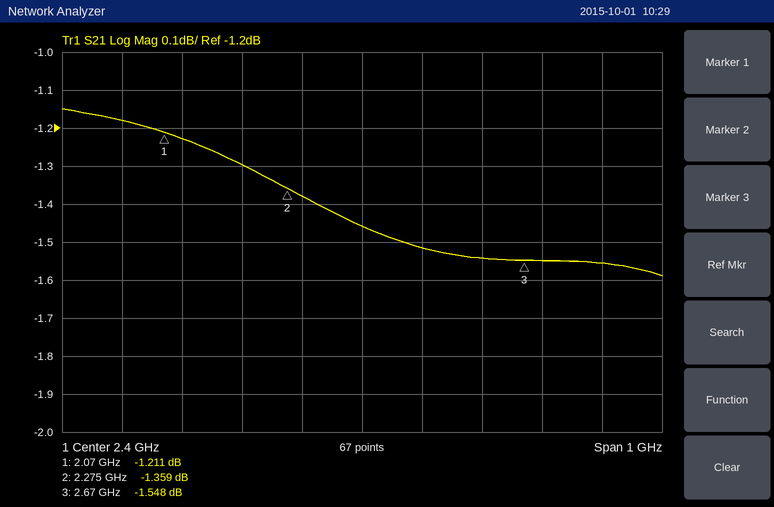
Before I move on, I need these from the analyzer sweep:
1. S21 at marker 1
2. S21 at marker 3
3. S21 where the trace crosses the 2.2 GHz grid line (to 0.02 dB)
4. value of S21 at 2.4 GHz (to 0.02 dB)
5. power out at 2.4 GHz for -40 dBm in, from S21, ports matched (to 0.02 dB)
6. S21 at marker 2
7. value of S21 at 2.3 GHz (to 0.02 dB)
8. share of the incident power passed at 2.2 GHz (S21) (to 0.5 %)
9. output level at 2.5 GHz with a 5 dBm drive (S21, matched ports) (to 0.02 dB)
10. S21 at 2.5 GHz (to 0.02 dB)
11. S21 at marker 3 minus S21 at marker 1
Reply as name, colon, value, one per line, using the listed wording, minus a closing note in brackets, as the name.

S21 at marker 1: -1.211 dB
S21 at marker 3: -1.548 dB
S21 where the trace crosses the 2.2 GHz grid line: -1.30 dB
value of S21 at 2.4 GHz: -1.46 dB
power out at 2.4 GHz for -40 dBm in, from S21, ports matched: -41.46 dBm
S21 at marker 2: -1.359 dB
value of S21 at 2.3 GHz: -1.38 dB
share of the incident power passed at 2.2 GHz (S21): 74.0 %
output level at 2.5 GHz with a 5 dBm drive (S21, matched ports): 3.48 dBm
S21 at 2.5 GHz: -1.52 dB
S21 at marker 3 minus S21 at marker 1: -0.337 dB
